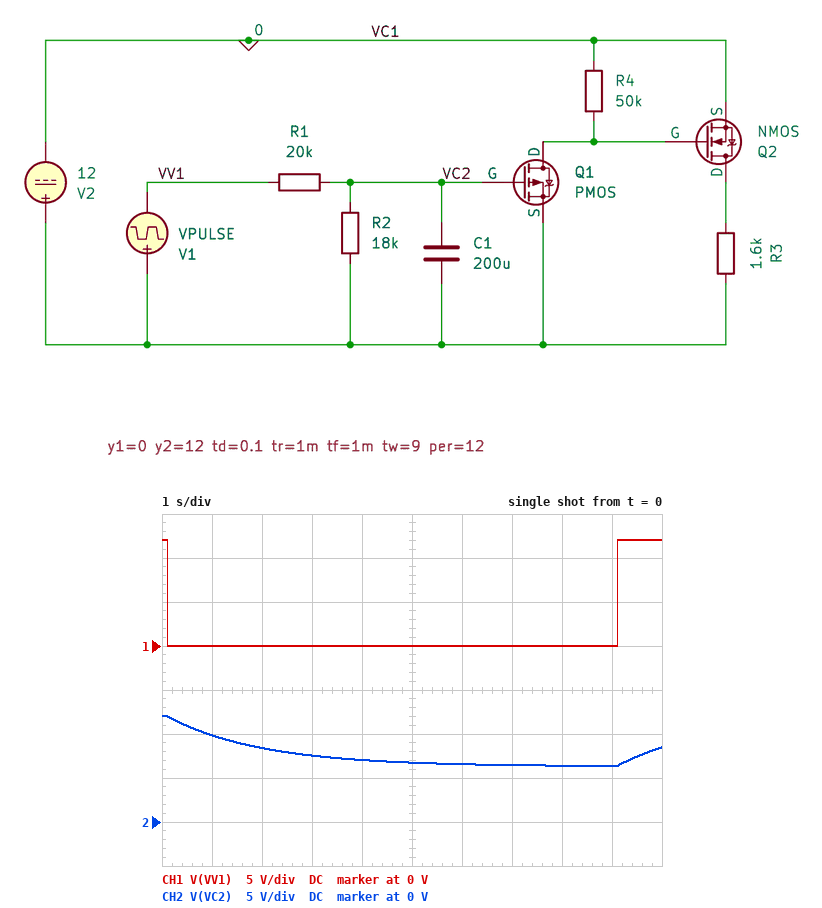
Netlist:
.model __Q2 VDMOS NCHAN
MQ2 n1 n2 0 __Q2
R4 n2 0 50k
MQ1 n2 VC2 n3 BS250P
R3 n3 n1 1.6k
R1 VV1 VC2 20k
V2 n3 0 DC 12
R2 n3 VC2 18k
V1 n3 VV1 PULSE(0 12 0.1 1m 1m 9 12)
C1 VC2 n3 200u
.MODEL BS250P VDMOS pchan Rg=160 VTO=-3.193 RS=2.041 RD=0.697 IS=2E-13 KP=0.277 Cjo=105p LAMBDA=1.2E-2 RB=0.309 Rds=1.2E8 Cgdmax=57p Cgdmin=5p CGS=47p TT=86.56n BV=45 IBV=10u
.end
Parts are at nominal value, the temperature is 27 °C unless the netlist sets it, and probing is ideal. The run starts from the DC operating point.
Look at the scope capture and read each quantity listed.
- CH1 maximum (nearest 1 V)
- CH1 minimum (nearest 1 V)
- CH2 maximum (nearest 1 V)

12 V
0 V
12 V
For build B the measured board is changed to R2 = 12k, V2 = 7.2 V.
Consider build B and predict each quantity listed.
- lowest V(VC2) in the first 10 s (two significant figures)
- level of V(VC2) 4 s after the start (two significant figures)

2.7 V
3.0 V
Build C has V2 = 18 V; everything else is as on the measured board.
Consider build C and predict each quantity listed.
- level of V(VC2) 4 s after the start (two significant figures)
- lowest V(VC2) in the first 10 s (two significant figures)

13 V
12 V
